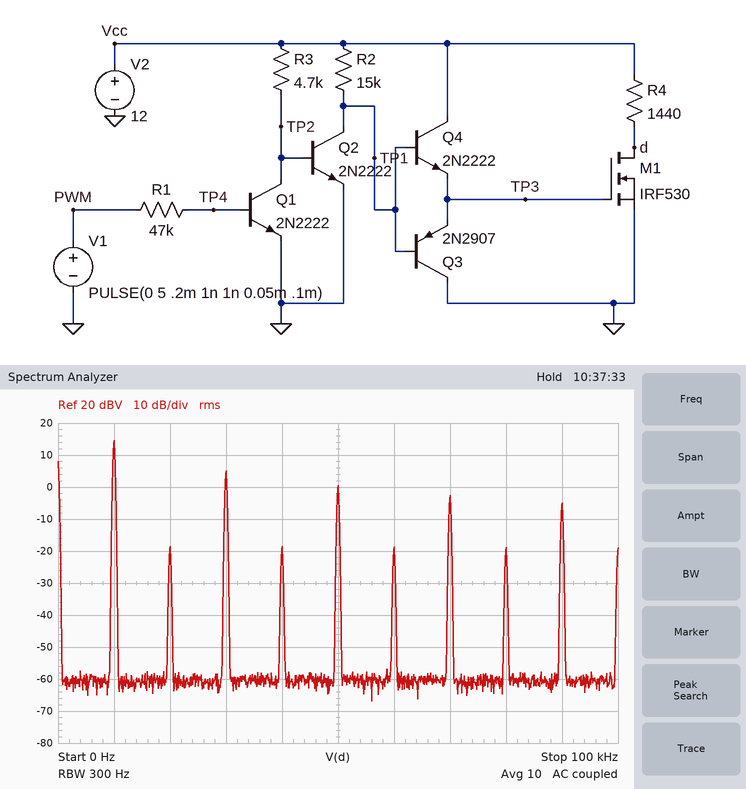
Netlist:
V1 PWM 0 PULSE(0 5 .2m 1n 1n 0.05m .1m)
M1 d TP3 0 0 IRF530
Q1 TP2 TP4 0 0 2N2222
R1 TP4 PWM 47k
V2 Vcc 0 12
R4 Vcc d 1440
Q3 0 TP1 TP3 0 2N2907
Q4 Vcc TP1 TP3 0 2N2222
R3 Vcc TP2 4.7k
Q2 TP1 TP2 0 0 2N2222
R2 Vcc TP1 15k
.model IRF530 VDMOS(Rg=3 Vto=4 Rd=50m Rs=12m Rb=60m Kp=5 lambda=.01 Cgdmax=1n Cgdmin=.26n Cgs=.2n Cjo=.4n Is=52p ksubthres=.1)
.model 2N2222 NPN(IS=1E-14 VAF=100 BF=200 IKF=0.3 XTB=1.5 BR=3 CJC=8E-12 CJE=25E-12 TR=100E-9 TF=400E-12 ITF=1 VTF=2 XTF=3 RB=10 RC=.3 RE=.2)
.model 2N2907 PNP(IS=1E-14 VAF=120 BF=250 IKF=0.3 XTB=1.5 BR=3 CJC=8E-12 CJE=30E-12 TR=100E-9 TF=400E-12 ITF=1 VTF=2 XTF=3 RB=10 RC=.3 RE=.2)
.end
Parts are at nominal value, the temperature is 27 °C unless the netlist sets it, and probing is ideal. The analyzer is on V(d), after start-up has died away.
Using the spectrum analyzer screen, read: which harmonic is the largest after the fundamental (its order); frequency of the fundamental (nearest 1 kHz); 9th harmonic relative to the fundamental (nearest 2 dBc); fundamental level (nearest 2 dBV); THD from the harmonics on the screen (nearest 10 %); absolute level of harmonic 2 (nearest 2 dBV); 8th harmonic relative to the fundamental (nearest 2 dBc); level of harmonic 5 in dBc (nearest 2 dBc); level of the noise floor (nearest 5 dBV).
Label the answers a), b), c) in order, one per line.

a) 3
b) 10 kHz
c) -20 dBc
d) 14 dBV
e) 40 %
f) -18 dBV
g) -34 dBc
h) -14 dBc
i) -60 dBV
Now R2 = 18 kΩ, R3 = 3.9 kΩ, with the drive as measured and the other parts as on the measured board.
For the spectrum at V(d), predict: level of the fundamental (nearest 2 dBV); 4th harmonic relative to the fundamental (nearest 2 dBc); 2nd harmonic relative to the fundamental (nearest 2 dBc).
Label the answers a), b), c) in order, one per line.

a) 14 dBV
b) -36 dBc
c) -36 dBc
